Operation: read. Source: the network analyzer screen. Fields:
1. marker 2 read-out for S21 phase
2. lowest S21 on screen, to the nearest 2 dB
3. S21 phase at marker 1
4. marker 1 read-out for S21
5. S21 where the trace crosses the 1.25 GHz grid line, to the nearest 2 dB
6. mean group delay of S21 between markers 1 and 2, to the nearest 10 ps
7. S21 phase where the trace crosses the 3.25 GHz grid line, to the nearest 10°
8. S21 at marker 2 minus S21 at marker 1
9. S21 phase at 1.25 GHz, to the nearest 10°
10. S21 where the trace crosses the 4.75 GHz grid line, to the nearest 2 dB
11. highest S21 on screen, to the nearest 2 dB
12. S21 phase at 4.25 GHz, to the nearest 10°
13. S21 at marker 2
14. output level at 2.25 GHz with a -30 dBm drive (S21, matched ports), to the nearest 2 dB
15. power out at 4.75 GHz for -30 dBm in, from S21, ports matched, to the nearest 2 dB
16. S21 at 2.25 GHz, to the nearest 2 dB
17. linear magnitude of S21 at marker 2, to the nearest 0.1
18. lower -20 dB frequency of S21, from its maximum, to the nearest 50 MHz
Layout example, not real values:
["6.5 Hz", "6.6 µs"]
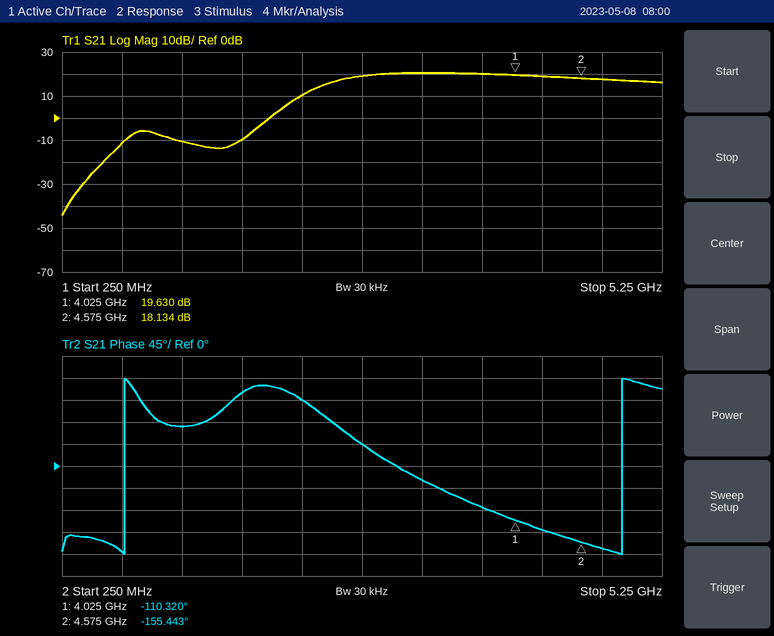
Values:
["-155.443°", "-44 dB", "-110.320°", "19.630 dB", "-10 dB", "230 ps", "-30°", "-1.496 dB", "80°", "18 dB", "20 dB", "-130°", "18.134 dB", "-20 dBm", "-12 dBm", "10 dB", "8.1", "2.00 GHz"]
